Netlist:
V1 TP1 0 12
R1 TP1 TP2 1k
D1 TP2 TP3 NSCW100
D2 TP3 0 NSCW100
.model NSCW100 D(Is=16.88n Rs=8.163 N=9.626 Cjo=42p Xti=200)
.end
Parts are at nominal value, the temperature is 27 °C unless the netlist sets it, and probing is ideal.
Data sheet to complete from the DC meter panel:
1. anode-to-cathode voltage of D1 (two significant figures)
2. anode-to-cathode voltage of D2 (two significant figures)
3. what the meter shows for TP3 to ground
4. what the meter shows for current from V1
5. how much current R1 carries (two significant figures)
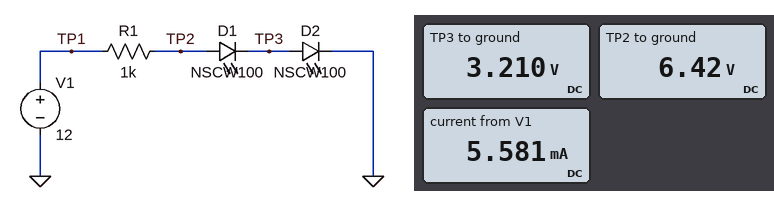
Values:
3.2 V
3.2 V
3.210 V
5.581 mA
5.6 mA
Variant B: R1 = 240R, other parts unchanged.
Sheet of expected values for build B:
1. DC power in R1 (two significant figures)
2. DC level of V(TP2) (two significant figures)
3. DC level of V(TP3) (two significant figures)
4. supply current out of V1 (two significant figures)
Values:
93 mW
7.3 V
3.6 V
20 mA
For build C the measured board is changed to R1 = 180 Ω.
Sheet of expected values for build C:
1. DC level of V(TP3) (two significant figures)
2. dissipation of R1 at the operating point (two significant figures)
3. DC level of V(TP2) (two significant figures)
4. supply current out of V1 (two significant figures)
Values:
3.7 V
110 mW
7.5 V
25 mA
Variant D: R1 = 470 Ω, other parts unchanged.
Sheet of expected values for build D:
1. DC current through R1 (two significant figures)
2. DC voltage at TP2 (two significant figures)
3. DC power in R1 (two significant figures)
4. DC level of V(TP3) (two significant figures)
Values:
11 mA
6.8 V
57 mW
3.4 V
